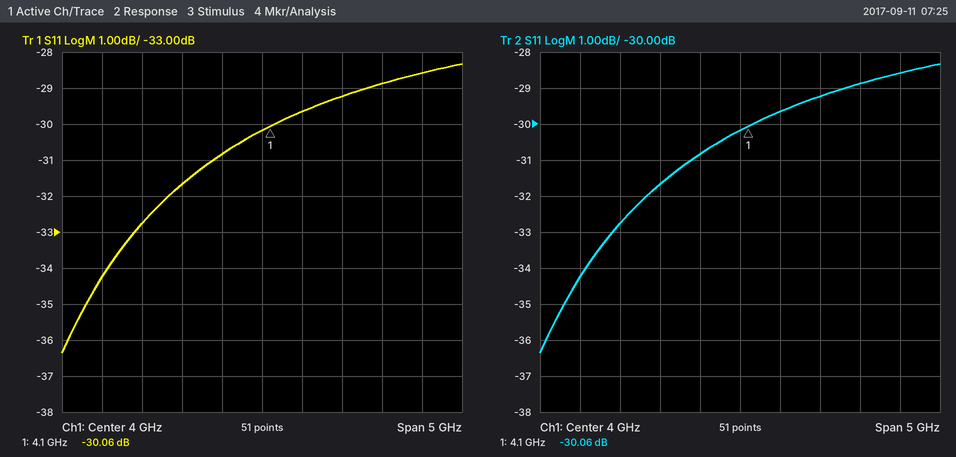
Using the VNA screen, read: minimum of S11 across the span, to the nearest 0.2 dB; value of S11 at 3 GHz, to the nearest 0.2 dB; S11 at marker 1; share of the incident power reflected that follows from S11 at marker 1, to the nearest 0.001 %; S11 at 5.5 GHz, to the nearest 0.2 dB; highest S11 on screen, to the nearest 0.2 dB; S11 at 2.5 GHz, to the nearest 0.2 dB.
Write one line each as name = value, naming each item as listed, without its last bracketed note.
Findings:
minimum of S11 across the span, to the nearest 0.2 dB = -36.4 dB
value of S11 at 3 GHz, to the nearest 0.2 dB = -31.6 dB
S11 at marker 1 = -30.06 dB
share of the incident power reflected that follows from S11 at marker 1, to the nearest 0.001 % = 0.099 %
S11 at 5.5 GHz, to the nearest 0.2 dB = -28.8 dB
highest S11 on screen, to the nearest 0.2 dB = -28.4 dB
S11 at 2.5 GHz, to the nearest 0.2 dB = -32.8 dB
